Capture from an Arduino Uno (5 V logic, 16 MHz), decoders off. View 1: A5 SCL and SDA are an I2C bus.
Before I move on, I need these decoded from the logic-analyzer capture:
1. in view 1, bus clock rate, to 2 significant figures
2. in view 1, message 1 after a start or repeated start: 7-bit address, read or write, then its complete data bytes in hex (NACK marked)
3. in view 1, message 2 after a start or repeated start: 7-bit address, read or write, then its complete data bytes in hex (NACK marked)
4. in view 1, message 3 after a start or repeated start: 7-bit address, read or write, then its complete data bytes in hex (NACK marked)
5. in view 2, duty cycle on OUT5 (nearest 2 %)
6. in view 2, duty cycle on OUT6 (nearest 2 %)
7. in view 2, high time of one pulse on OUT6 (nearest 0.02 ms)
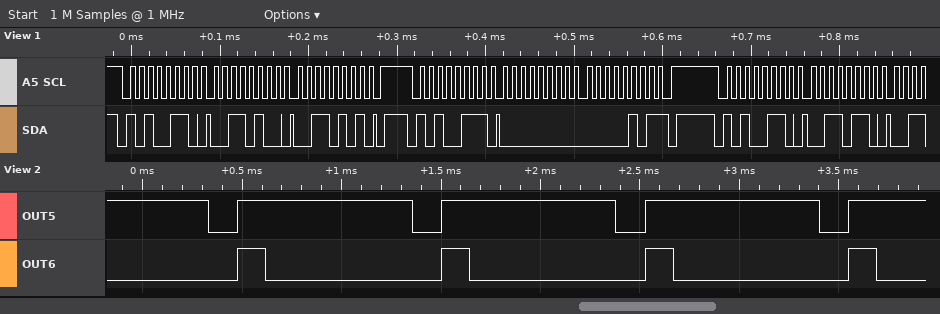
100 kHz
0x53 write: 34 35
0x53 read: 00 05 NACK
0x53 write: 36
86 %
14 %
0.14 ms
